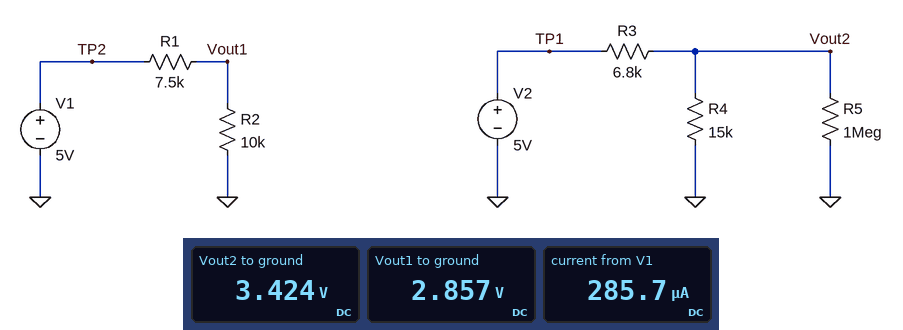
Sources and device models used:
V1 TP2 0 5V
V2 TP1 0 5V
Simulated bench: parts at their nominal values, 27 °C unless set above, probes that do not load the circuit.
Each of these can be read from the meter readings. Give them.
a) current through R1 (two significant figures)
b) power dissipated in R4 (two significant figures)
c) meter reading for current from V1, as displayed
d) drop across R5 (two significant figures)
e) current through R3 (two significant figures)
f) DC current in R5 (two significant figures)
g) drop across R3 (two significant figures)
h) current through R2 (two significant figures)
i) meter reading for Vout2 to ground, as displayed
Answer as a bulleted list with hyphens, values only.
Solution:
- 290 µA
- 780 µW
- 285.7 µA
- 3.4 V
- 230 µA
- 3.4 µA
- 1.6 V
- 290 µA
- 3.424 V
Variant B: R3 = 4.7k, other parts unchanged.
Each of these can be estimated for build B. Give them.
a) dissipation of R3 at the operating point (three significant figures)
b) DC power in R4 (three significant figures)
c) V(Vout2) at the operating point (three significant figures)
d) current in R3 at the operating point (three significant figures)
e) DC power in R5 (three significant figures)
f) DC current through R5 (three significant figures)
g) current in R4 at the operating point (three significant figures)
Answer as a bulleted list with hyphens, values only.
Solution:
- 310 µW
- 959 µW
- 3.79 V
- 257 µA
- 14.4 µW
- 3.79 µA
- 253 µA
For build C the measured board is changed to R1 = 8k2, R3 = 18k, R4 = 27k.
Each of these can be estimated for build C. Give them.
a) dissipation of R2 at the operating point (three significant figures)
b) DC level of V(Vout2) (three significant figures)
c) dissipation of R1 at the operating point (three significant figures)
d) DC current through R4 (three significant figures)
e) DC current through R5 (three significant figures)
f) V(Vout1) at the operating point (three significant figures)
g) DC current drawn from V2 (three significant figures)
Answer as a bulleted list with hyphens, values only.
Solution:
- 755 µW
- 2.97 V
- 619 µW
- 110 µA
- 2.97 µA
- 2.75 V
- 113 µA
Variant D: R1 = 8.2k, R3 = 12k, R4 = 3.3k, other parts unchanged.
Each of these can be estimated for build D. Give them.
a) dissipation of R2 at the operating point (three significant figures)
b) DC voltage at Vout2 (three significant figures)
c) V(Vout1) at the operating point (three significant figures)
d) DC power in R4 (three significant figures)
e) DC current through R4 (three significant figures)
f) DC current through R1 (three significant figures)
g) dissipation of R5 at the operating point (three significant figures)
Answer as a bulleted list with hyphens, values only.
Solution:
- 755 µW
- 1.08 V
- 2.75 V
- 351 µW
- 326 µA
- 275 µA
- 1.16 µW
